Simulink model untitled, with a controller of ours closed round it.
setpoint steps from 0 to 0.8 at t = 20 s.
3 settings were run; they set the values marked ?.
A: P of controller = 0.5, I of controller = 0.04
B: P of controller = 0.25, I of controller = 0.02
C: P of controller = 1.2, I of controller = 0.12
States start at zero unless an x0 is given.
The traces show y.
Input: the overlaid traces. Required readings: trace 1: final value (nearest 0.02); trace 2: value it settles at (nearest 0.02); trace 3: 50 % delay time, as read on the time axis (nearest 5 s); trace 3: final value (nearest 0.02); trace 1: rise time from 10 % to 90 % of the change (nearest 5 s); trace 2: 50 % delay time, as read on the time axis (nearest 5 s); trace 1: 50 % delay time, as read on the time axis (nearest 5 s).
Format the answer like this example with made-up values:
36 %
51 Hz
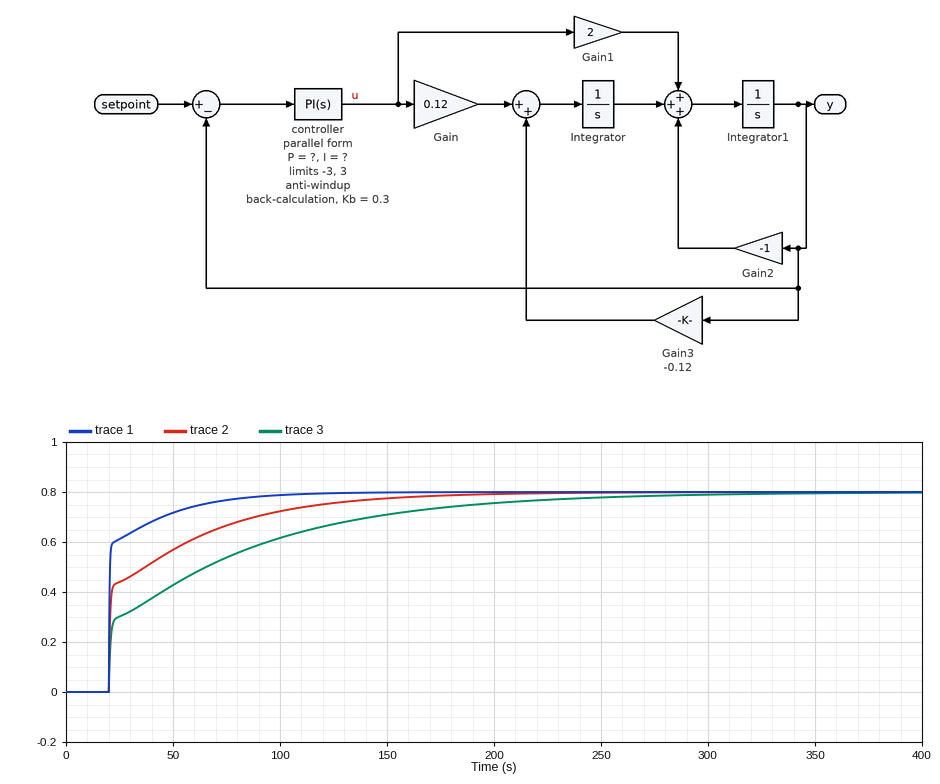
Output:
0.80
0.80
45 s
0.80
30 s
20 s
20 s
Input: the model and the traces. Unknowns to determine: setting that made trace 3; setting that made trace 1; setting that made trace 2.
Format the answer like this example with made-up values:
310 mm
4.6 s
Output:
B
C
A
